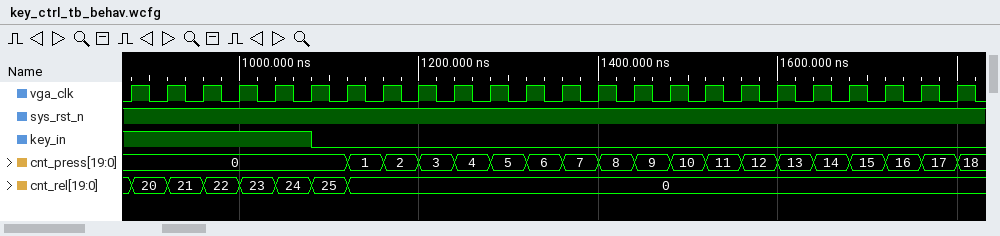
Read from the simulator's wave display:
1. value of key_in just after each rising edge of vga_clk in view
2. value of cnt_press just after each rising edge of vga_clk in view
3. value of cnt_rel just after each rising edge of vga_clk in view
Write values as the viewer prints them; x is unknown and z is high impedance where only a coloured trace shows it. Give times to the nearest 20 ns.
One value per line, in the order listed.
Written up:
1 1 1 1 1 0 0 0 0 0 0 0 0 0 0 0 0 0 0 0 0 0 0 0
0, 0, 0, 0, 0, 0, 1, 2, 3, 4, 5, 6, 7, 8, 9, 10, 11, 12, 13, 14, 15, 16, 17, 18
20, 21, 22, 23, 24, 25, 0, 0, 0, 0, 0, 0, 0, 0, 0, 0, 0, 0, 0, 0, 0, 0, 0, 0
